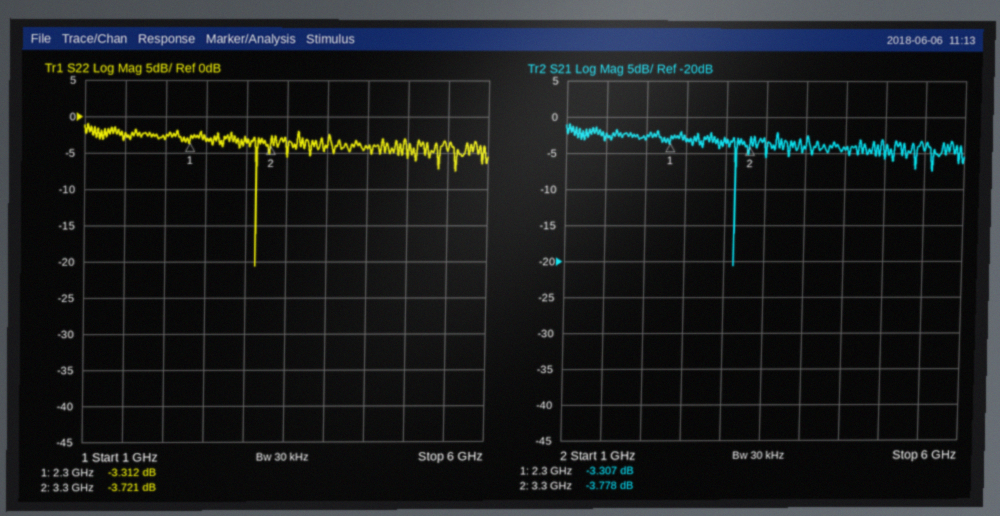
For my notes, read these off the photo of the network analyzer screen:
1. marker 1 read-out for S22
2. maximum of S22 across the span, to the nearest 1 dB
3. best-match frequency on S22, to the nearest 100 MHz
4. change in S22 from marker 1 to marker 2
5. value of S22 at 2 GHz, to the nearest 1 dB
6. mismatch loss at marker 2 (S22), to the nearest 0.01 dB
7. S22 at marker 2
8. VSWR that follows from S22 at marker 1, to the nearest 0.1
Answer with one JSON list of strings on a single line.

["-3.312 dB", "-1 dB", "3.1 GHz", "-0.409 dB", "-3 dB", "2.40 dB", "-3.721 dB", "5.3"]
